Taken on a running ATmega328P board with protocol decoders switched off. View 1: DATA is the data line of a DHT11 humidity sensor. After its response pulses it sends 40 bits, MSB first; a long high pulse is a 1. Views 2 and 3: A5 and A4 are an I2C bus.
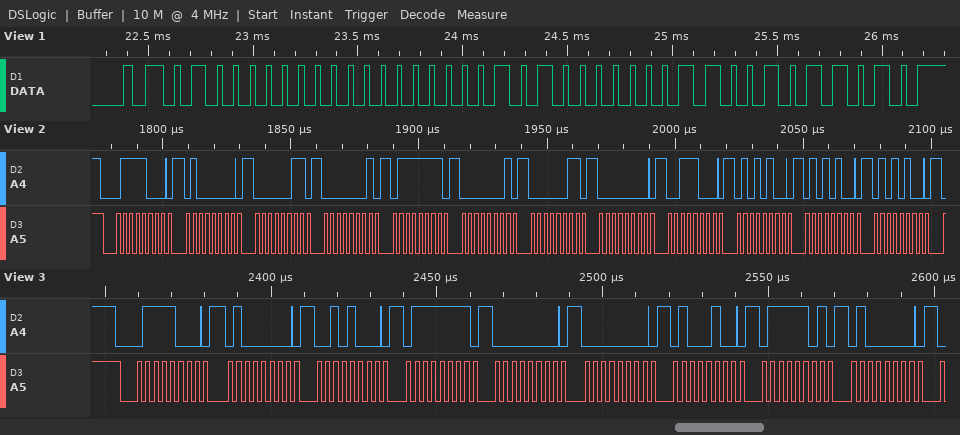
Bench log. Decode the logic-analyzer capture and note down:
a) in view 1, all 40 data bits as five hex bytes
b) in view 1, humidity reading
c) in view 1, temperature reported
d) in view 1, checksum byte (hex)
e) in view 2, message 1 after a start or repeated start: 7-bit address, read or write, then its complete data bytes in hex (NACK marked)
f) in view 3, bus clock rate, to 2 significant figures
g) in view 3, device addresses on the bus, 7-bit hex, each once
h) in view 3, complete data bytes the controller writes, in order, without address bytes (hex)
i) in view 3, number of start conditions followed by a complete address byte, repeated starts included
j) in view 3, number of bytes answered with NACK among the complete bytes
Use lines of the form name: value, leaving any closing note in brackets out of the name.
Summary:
in view 1, all 40 data bits as five hex bytes: 40 00 14 06 5A
in view 1, humidity reading: 64 %
in view 1, temperature reported: 20.6 °C
in view 1, checksum byte: 0x5A
in view 2, message 1 after a start or repeated start: 7-bit address, read or write, then its complete data bytes in hex: 0x3C write: 40 03 01 7F 01 03 00 38 54 54 54
in view 3, bus clock rate, to 2 significant figures: 400 kHz
in view 3, device addresses on the bus, 7-bit hex, each once: 0x3C
in view 3, complete data bytes the controller writes, in order, without address bytes: 40 28 7F 00 00 44 7D 40
in view 3, number of start conditions followed by a complete address byte, repeated starts included: 1
in view 3, number of bytes answered with NACK among the complete bytes: 0
